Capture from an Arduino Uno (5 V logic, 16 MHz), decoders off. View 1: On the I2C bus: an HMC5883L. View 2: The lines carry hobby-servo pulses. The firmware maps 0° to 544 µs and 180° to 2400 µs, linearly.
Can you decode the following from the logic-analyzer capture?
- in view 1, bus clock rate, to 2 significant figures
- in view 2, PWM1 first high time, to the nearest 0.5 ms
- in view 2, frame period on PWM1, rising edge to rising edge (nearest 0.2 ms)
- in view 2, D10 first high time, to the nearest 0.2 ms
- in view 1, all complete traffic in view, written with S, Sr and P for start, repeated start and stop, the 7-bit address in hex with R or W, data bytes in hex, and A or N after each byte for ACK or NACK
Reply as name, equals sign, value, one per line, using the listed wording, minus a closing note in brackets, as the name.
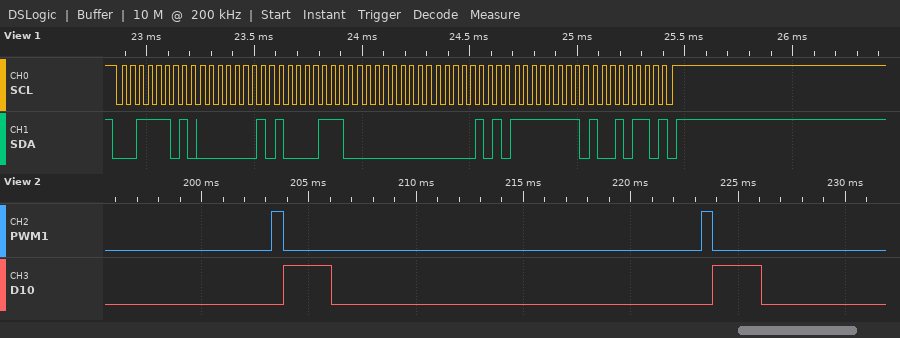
in view 1, bus clock rate, to 2 significant figures = 25 kHz
in view 2, PWM1 first high time, to the nearest 0.5 ms = 0.5 ms
in view 2, frame period on PWM1, rising edge to rising edge = 20.0 ms
in view 2, D10 first high time, to the nearest 0.2 ms = 2.2 ms
in view 1, all complete traffic in view, written with S, Sr and P for start, repeated start and stop, the 7-bit address in hex with R or W, data bytes in hex, and A or N after each byte for ACK or NACK = S 1ER A 01 A 87 A 00 A 05 A FF A 96 N P
